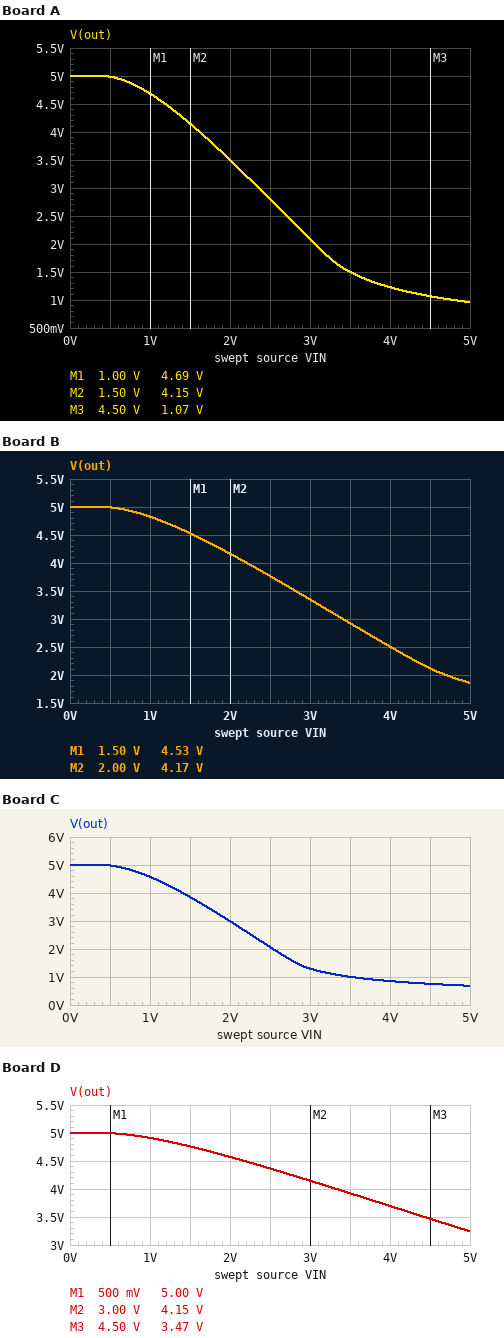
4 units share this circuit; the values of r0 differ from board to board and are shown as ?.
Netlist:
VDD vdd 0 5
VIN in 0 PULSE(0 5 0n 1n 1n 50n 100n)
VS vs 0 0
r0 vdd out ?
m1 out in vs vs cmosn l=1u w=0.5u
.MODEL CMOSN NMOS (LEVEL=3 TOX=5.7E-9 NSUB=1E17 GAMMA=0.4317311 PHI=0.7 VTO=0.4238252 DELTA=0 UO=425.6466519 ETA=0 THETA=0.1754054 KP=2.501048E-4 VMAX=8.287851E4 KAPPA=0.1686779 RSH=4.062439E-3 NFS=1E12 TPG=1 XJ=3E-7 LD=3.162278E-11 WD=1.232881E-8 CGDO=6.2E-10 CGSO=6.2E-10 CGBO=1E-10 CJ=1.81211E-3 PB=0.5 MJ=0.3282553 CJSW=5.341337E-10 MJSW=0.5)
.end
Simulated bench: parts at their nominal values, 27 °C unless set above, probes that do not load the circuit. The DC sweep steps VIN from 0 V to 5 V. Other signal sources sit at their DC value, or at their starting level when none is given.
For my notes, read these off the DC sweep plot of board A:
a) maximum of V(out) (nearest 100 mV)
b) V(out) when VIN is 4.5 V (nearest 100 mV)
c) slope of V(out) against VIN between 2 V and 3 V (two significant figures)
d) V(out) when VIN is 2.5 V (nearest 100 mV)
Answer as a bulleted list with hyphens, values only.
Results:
- 5.0 V
- 1.1 V
- -1.4 V/V
- 2.8 V
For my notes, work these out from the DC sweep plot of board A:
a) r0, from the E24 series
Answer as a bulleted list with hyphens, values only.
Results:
- 20 kΩ
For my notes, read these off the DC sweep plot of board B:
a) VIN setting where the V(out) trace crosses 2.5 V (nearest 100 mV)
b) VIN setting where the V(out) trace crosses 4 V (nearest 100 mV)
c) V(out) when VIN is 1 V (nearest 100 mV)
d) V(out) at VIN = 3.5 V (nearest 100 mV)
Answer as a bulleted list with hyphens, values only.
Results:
- 4.0 V
- 2.2 V
- 4.8 V
- 2.9 V
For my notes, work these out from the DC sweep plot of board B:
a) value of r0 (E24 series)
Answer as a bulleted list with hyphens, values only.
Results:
- 11 kΩ
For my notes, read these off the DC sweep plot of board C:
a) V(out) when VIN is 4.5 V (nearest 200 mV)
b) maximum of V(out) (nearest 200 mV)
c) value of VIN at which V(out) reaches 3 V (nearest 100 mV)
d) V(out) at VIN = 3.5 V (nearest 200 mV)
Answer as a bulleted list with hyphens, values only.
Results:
- 800 mV
- 5.0 V
- 2.0 V
- 1.0 V
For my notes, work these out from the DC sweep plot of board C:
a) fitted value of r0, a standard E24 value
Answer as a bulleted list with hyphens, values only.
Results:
- 27 kΩ
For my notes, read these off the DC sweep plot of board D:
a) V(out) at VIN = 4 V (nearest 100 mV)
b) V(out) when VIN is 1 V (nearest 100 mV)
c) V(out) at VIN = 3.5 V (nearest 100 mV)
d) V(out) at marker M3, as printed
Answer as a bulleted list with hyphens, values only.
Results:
- 3.7 V
- 4.9 V
- 3.9 V
- 3.47 V
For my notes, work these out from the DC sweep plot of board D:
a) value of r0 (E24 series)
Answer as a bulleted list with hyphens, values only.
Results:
- 5.6 kΩ
